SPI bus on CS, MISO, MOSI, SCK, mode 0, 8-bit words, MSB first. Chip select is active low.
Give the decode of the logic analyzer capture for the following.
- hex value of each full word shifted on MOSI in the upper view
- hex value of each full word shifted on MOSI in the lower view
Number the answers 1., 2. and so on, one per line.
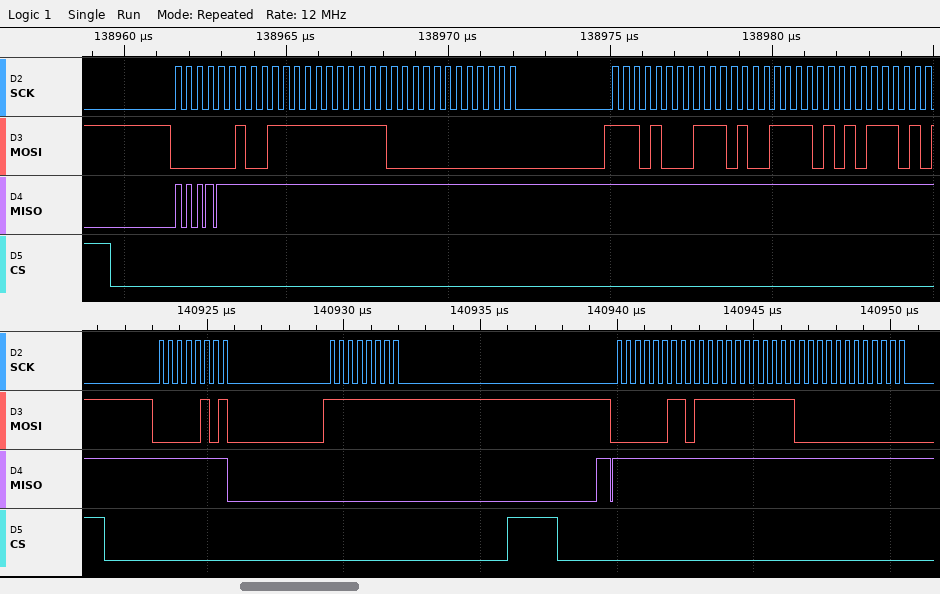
1. 02, 7F, F0, 00, E8, E9, EA
2. 05, FF, 03, 7F, F0, 00
